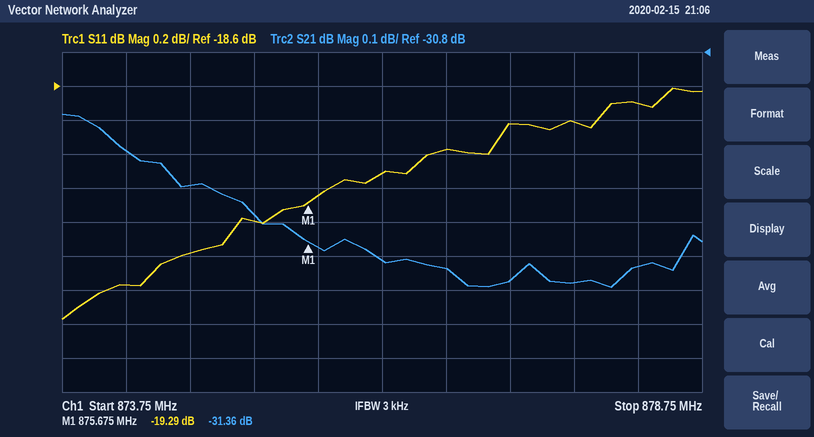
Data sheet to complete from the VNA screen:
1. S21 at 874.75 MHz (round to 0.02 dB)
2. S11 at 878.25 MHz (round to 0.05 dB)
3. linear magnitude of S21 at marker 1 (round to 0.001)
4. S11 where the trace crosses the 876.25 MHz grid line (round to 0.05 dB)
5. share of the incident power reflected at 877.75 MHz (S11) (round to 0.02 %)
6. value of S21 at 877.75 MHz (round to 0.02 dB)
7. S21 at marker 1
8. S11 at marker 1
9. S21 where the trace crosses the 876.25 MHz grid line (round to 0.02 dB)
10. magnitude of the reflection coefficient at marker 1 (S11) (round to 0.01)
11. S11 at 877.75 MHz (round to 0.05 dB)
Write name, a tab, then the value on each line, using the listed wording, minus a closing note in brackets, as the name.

S21 at 874.75 MHz	-31.20 dB
S11 at 878.25 MHz	-18.70 dB
linear magnitude of S21 at marker 1	0.027
S11 where the trace crosses the 876.25 MHz grid line	-19.10 dB
share of the incident power reflected at 877.75 MHz (S11)	1.32 %
value of S21 at 877.75 MHz	-31.48 dB
S21 at marker 1	-31.36 dB
S11 at marker 1	-19.29 dB
S21 where the trace crosses the 876.25 MHz grid line	-31.42 dB
magnitude of the reflection coefficient at marker 1 (S11)	0.11
S11 at 877.75 MHz	-18.80 dB
